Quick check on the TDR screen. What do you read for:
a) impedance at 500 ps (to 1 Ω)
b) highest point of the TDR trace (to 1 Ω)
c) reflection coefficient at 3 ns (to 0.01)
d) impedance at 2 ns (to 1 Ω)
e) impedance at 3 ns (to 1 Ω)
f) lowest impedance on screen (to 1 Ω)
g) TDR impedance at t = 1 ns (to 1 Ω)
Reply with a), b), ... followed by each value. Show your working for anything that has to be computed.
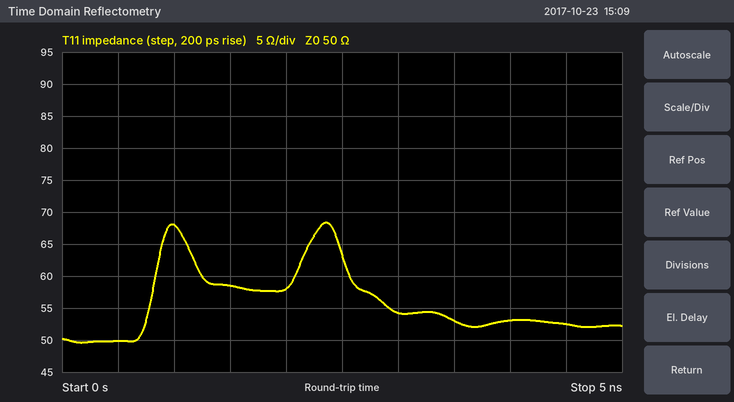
a) 50 Ω
b) 68 Ω
c) (54 − 50)/(54 + 50) ≈ +0.04
d) 58 Ω
e) 54 Ω
f) 50 Ω
g) 68 Ω
